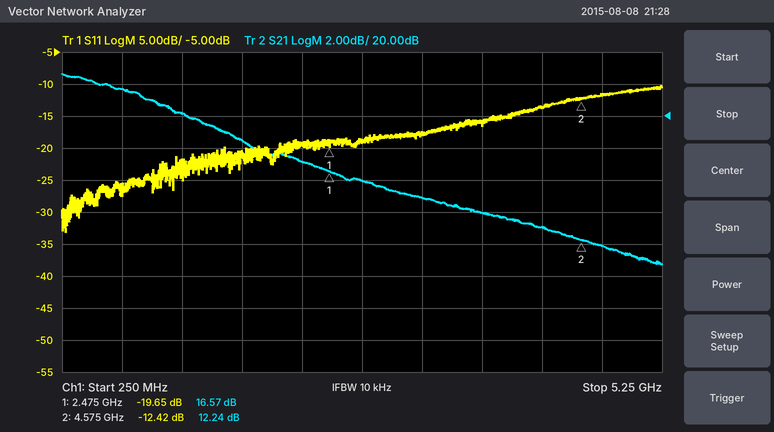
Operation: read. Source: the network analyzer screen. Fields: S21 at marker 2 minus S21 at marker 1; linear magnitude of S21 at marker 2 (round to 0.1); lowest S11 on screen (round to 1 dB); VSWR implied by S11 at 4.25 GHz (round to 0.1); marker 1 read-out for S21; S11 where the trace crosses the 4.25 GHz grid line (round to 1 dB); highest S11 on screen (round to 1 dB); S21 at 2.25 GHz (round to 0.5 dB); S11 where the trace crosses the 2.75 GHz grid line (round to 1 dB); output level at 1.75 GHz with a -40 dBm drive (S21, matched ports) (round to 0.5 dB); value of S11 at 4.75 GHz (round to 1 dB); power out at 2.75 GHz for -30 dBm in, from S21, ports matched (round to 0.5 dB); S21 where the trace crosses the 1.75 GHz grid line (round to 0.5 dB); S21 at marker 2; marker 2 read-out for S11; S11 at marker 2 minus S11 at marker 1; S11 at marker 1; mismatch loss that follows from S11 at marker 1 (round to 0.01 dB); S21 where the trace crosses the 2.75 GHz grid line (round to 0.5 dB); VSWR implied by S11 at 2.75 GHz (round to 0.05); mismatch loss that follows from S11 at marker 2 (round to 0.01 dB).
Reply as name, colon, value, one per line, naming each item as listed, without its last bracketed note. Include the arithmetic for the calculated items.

S21 at marker 2 minus S21 at marker 1: 12.24 − (16.57) = -4.33 dB
linear magnitude of S21 at marker 2: 10^(12.24/20) ≈ 4.1
lowest S11 on screen: -33 dB
VSWR implied by S11 at 4.25 GHz: |Γ| = 10^(-14/20) = 0.1995; VSWR = (1 + 0.1995)/(1 − 0.1995) ≈ 1.5
marker 1 read-out for S21: 16.57 dB
S11 where the trace crosses the 4.25 GHz grid line: -14 dB
highest S11 on screen: -10 dB
S21 at 2.25 GHz: 17.0 dB
S11 where the trace crosses the 2.75 GHz grid line: -19 dB
output level at 1.75 GHz with a -40 dBm drive (S21, matched ports): -40 dBm + (18.5 dB) = -21.5 dBm
value of S11 at 4.75 GHz: -12 dB
power out at 2.75 GHz for -30 dBm in, from S21, ports matched: -30 dBm + (16.0 dB) = -14.0 dBm
S21 where the trace crosses the 1.75 GHz grid line: 18.5 dB
S21 at marker 2: 12.24 dB
marker 2 read-out for S11: -12.42 dB
S11 at marker 2 minus S11 at marker 1: -12.42 − (-19.65) = 7.23 dB
S11 at marker 1: -19.65 dB
mismatch loss that follows from S11 at marker 1: −10 log10(1 − 10^(-19.65/10)) ≈ 0.05 dB
S21 where the trace crosses the 2.75 GHz grid line: 16.0 dB
VSWR implied by S11 at 2.75 GHz: |Γ| = 10^(-19/20) = 0.1122; VSWR = (1 + 0.1122)/(1 − 0.1122) ≈ 1.25
mismatch loss that follows from S11 at marker 2: −10 log10(1 − 10^(-12.42/10)) ≈ 0.26 dB
